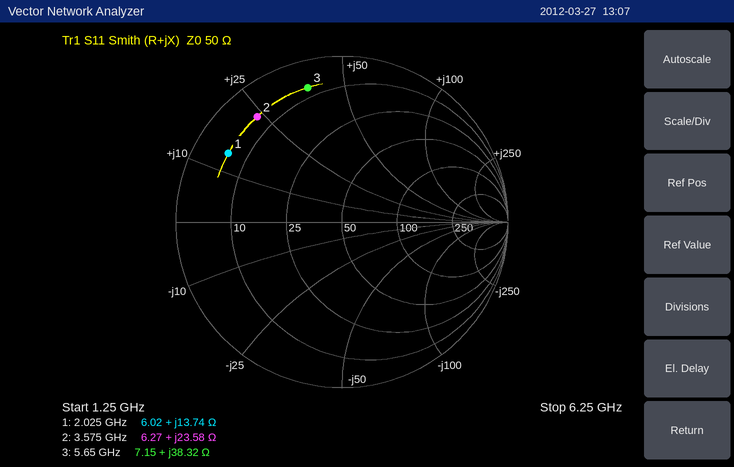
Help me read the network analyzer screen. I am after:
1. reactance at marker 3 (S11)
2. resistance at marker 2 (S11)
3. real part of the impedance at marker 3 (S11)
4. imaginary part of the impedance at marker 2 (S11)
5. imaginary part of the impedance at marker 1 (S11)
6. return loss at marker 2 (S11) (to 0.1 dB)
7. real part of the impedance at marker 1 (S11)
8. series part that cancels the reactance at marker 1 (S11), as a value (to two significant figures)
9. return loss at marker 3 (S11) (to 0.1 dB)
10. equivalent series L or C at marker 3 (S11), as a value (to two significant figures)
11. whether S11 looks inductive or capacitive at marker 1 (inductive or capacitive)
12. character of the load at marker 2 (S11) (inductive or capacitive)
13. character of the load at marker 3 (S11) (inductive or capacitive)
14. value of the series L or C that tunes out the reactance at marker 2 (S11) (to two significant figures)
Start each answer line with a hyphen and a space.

- +38.32 Ω
- 6.27 Ω
- 7.15 Ω
- +23.58 Ω
- +13.74 Ω
- 1.8 dB
- 6.02 Ω
- 5.7 pF
- 1.6 dB
- 1.1 nH
- inductive
- inductive
- inductive
- 1.9 pF
